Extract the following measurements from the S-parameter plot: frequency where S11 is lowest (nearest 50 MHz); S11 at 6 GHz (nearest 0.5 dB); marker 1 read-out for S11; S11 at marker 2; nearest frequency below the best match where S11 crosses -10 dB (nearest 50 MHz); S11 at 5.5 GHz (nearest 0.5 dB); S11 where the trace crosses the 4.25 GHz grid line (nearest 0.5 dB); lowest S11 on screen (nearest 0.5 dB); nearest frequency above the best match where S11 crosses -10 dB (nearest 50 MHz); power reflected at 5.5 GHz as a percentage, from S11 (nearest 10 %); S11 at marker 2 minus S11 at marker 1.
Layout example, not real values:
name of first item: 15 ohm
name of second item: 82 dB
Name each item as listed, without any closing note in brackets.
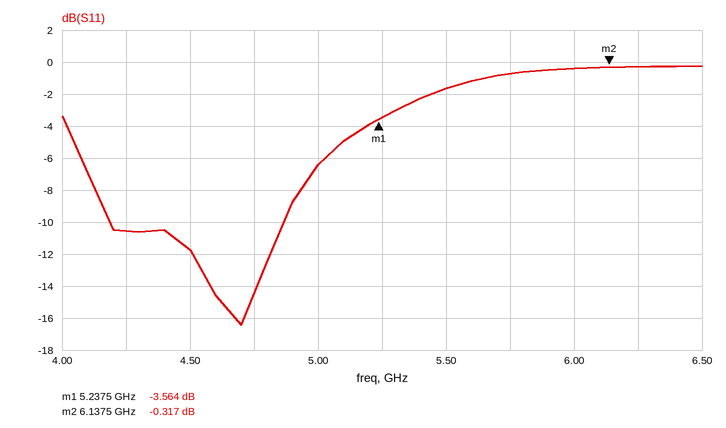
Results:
frequency where S11 is lowest: 4.70 GHz
S11 at 6 GHz: -0.5 dB
marker 1 read-out for S11: -3.564 dB
S11 at marker 2: -0.317 dB
nearest frequency below the best match where S11 crosses -10 dB: 4.20 GHz
S11 at 5.5 GHz: -1.5 dB
S11 where the trace crosses the 4.25 GHz grid line: -10.5 dB
lowest S11 on screen: -16.5 dB
nearest frequency above the best match where S11 crosses -10 dB: 4.85 GHz
power reflected at 5.5 GHz as a percentage, from S11: 70 %
S11 at marker 2 minus S11 at marker 1: 3.247 dB
